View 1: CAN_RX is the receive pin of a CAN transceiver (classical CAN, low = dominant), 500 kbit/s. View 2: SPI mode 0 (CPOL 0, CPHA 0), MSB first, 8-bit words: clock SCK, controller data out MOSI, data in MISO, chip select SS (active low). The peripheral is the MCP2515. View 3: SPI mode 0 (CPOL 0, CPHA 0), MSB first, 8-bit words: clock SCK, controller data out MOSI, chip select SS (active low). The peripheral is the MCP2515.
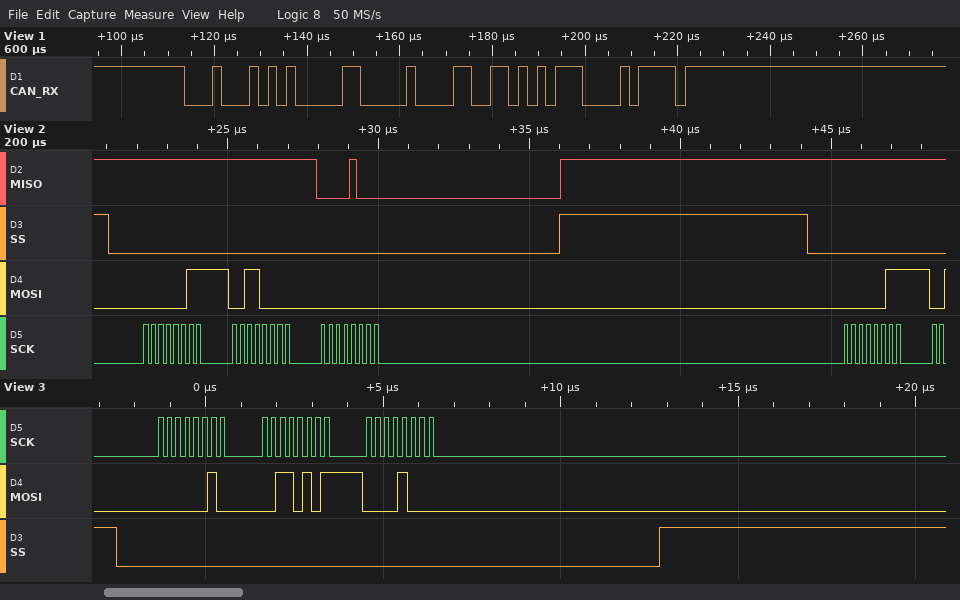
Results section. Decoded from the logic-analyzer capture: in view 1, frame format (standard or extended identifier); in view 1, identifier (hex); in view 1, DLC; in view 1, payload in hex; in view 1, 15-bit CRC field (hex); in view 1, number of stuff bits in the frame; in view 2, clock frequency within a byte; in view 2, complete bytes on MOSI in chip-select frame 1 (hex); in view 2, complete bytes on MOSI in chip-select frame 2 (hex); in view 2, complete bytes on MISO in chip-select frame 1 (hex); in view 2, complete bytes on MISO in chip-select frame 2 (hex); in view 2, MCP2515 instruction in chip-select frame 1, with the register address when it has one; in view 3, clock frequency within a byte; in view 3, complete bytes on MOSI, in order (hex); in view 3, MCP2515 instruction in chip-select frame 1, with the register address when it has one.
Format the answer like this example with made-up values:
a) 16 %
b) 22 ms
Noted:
a) standard
b) 0x115
c) 2
d) 00 CD
e) 0x2E17
f) 2
g) 4 MHz
h) 0x03 0x30 0x00
i) 0x03
j) 0xFF 0xFF 0x08
k) 0xFF
l) READ 0x30
m) 4 MHz
n) 02 35 08
o) WRITE 0x35
